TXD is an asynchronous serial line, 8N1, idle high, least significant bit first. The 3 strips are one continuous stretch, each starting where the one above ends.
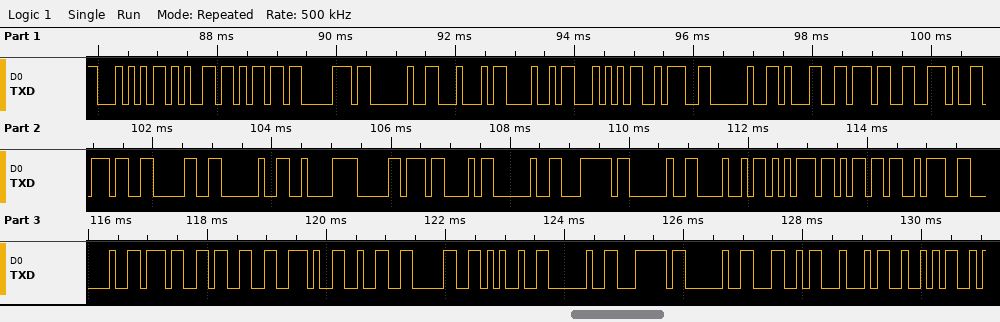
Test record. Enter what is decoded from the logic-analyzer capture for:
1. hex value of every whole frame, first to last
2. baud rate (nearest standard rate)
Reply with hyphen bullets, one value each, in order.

- 54 65 6D 70 20 44 48 54 3A 20 31 37 2E 37 30 20 C2 B0 43 20 7C 20 48 75 6D 3A 20 37 33 2E 32 30 25 20 7C 20 4C 44 52
- 9600 baud
